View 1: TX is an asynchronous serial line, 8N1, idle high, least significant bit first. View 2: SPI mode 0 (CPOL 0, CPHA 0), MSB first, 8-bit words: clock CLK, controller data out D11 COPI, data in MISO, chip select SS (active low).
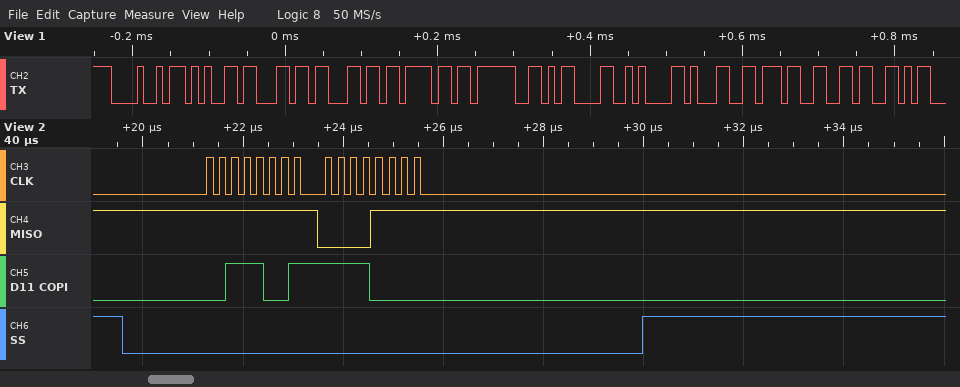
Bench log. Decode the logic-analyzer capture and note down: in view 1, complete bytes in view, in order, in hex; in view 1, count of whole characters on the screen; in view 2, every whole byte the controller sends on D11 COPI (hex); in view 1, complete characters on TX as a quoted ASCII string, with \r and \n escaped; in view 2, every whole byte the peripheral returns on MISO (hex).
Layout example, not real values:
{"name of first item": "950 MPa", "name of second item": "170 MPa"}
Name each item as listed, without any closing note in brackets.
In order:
{"in view 1, complete bytes in view, in order, in hex": "48 65 6C 6C 6F 3F 0D 0A 31 37 36", "in view 1, count of whole characters on the screen": "11", "in view 2, every whole byte the controller sends on D11 COPI": "39 F0", "in view 1, complete characters on TX as a quoted ASCII string, with \\r and \\n escaped": "\"Hello?\\r\\n176\"", "in view 2, every whole byte the peripheral returns on MISO": "FF 0F"}
